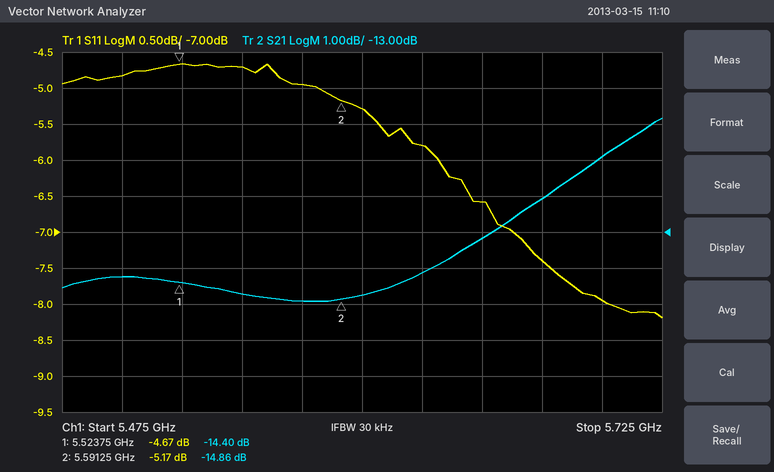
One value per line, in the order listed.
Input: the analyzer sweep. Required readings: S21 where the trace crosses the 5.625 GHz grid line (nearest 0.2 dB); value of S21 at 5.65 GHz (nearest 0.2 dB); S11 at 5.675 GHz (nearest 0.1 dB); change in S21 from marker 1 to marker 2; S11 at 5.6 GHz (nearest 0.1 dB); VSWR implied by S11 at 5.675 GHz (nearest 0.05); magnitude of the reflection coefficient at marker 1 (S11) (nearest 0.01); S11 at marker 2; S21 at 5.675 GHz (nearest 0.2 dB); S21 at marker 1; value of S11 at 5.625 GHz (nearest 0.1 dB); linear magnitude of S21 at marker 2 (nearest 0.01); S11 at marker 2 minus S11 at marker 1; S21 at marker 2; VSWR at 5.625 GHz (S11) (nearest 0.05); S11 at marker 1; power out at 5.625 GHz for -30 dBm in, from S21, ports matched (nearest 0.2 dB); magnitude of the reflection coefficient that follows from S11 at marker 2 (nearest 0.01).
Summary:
-14.2 dB
-13.2 dB
-7.4 dB
-0.46 dB
-5.3 dB
2.50
0.58
-5.17 dB
-12.0 dB
-14.40 dB
-5.8 dB
0.18
-0.50 dB
-14.86 dB
3.10
-4.67 dB
-44.2 dBm
0.55
